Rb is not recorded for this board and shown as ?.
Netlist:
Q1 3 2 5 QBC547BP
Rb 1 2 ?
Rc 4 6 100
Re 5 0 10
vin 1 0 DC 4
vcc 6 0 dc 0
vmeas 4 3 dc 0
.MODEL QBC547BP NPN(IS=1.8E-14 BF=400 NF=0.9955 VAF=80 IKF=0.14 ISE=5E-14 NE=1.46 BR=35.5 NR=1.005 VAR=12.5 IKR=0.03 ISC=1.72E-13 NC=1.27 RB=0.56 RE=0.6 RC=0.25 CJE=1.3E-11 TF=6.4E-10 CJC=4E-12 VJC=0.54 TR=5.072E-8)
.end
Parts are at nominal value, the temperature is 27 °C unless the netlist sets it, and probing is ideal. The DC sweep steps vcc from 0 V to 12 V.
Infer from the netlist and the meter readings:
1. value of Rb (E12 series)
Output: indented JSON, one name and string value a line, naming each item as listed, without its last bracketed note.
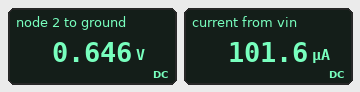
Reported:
{
  "value of Rb": "33 kΩ"
}
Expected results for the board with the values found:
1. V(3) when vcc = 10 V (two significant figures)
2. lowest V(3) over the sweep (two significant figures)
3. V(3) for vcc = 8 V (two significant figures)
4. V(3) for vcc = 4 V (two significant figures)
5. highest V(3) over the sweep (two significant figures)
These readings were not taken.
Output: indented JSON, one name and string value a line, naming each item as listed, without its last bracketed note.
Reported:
{
  "V(3) when vcc = 10 V": "7.3 V",
  "lowest V(3) over the sweep": "-2.1 mV",
  "V(3) for vcc = 8 V": "5.3 V",
  "V(3) for vcc = 4 V": "1.5 V",
  "highest V(3) over the sweep": "9.2 V"
}
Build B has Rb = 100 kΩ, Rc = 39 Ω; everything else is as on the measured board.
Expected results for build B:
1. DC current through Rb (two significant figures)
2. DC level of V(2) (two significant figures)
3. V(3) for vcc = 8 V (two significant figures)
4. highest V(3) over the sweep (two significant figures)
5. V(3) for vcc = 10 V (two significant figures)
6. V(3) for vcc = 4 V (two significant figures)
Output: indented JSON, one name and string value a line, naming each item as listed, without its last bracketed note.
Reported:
{
  "DC current through Rb": "34 µA",
  "DC level of V(2)": "610 mV",
  "V(3) for vcc = 8 V": "7.6 V",
  "highest V(3) over the sweep": "12 V",
  "V(3) for vcc = 10 V": "9.6 V",
  "V(3) for vcc = 4 V": "3.6 V"
}
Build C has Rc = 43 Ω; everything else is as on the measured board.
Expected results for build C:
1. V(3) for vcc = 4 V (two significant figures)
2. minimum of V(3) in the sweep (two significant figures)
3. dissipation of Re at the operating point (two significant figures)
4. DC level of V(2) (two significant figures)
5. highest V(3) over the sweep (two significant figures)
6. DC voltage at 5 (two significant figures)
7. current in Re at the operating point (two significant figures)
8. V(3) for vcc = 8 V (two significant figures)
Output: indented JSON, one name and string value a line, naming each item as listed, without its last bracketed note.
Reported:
{
  "V(3) for vcc = 4 V": "2.9 V",
  "minimum of V(3) in the sweep": "-1.6 mV",
  "dissipation of Re at the operating point": "190 nW",
  "DC level of V(2)": "650 mV",
  "highest V(3) over the sweep": "11 V",
  "DC voltage at 5": "1.4 mV",
  "current in Re at the operating point": "140 µA",
  "V(3) for vcc = 8 V": "6.8 V"
}
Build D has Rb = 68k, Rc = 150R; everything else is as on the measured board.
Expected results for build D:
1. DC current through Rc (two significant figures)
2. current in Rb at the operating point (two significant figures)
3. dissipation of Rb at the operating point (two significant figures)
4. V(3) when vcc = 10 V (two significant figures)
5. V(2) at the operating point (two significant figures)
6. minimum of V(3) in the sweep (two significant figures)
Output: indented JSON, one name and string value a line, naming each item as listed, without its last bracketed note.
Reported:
{
  "DC current through Rc": "14 µA",
  "current in Rb at the operating point": "50 µA",
  "dissipation of Rb at the operating point": "170 µW",
  "V(3) when vcc = 10 V": "7.8 V",
  "V(2) at the operating point": "620 mV",
  "minimum of V(3) in the sweep": "-2.1 mV"
}
